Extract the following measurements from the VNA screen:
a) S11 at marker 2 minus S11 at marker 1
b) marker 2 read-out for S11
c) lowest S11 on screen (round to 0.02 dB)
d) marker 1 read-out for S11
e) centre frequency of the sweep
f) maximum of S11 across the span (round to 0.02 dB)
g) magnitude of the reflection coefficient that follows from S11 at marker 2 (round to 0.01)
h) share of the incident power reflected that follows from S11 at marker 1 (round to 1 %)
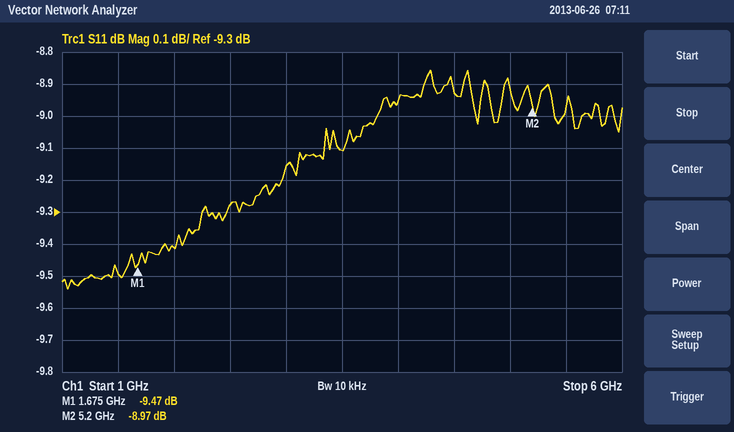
0.50 dB
-8.97 dB
-9.54 dB
-9.47 dB
3.5 GHz
-8.86 dB
0.36
11 %
